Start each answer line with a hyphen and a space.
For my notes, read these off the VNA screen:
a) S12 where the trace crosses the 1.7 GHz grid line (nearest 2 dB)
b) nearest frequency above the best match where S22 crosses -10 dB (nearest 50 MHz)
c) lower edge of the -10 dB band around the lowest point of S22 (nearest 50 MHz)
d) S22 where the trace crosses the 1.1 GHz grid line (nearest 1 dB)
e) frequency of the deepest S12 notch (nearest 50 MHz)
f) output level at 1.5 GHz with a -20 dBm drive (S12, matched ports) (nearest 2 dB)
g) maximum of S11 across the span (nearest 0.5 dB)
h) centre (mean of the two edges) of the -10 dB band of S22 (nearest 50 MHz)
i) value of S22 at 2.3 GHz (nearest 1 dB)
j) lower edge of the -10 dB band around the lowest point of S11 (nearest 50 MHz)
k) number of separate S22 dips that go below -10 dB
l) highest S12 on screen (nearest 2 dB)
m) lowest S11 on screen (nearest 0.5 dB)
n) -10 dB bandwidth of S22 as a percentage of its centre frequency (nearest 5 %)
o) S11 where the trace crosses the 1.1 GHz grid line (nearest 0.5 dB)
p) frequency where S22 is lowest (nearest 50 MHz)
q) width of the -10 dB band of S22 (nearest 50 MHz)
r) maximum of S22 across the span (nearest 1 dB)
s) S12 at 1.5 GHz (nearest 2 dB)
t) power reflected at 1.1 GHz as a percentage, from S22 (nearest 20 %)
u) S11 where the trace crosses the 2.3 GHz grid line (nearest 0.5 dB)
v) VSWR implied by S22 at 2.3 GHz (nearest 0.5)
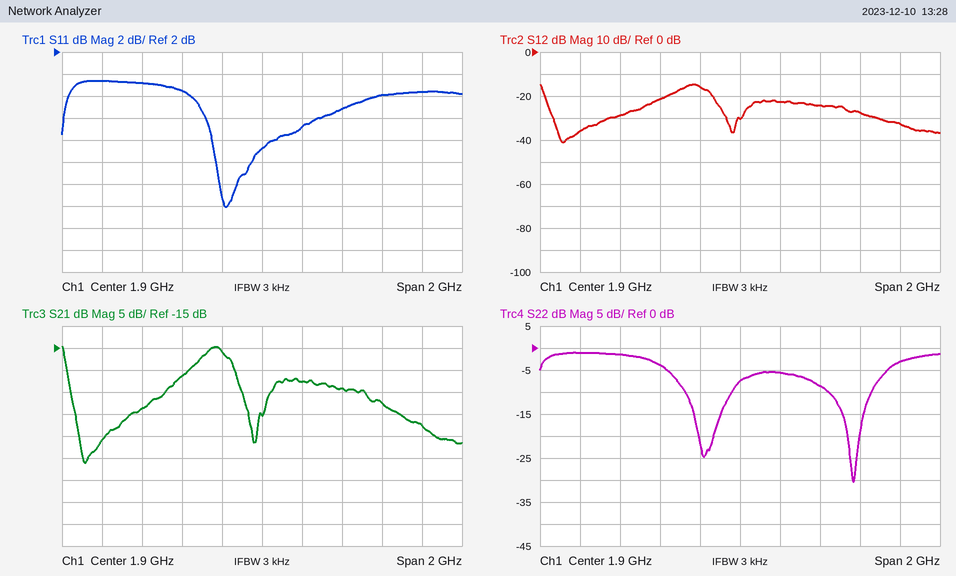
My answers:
- -16 dB
- 2.55 GHz
- 2.35 GHz
- -1 dB
- 1.00 GHz
- -42 dBm
- -0.5 dB
- 2.45 GHz
- -9 dB
- 1.70 GHz
- 2
- -14 dB
- -12.0 dB
- 10 %
- -0.5 dB
- 2.45 GHz
- 200 MHz
- -1 dB
- -22 dB
- 80 %
- -3.0 dB
- 2.0
